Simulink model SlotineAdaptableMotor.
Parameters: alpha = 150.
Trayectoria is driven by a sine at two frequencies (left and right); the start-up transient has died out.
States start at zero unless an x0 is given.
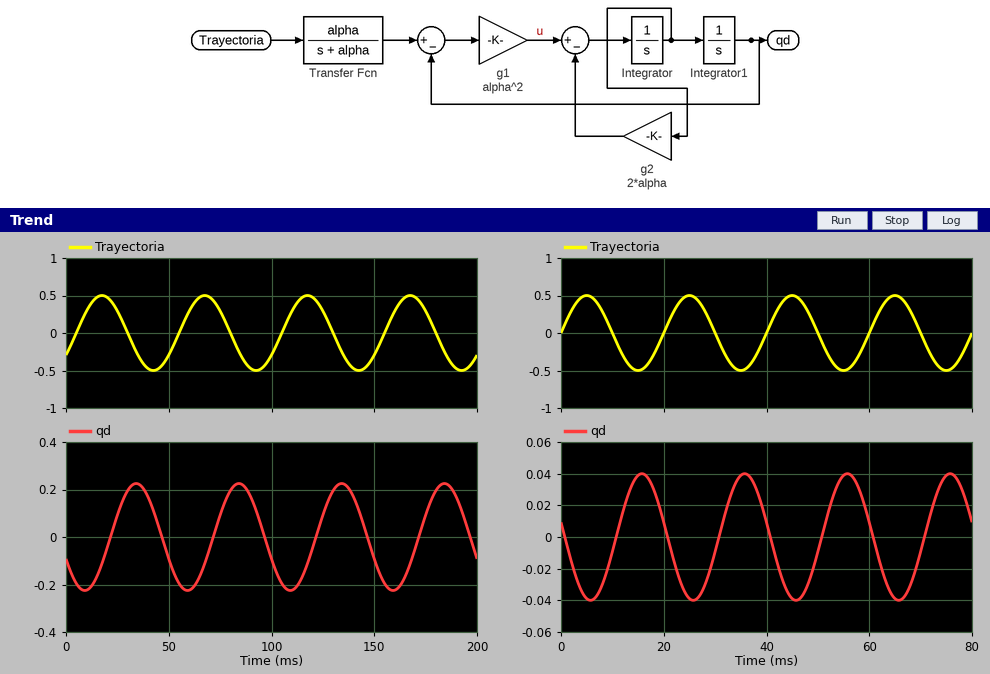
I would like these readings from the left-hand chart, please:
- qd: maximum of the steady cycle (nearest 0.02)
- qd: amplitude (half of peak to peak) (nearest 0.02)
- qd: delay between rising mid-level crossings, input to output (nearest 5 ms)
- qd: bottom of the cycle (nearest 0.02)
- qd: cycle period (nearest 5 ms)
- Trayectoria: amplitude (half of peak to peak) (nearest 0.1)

0.22
0.22
15 ms
-0.22
50 ms
0.5
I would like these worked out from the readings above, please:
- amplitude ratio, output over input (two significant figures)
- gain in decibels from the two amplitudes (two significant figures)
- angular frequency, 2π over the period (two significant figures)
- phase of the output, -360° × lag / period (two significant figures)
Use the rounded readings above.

0.44
-7.1 dB
0.13 rad/ms
-110°
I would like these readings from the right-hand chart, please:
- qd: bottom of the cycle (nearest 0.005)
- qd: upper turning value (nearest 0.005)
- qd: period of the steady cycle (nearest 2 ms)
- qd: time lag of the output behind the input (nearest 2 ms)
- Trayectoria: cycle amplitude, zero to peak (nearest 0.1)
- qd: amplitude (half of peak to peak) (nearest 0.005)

-0.040
0.040
20 ms
10 ms
0.5
0.040
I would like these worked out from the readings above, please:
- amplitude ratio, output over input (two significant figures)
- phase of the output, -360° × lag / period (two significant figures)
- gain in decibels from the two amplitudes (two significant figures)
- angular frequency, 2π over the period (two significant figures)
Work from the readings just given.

0.080
-180°
-22 dB
0.31 rad/ms
